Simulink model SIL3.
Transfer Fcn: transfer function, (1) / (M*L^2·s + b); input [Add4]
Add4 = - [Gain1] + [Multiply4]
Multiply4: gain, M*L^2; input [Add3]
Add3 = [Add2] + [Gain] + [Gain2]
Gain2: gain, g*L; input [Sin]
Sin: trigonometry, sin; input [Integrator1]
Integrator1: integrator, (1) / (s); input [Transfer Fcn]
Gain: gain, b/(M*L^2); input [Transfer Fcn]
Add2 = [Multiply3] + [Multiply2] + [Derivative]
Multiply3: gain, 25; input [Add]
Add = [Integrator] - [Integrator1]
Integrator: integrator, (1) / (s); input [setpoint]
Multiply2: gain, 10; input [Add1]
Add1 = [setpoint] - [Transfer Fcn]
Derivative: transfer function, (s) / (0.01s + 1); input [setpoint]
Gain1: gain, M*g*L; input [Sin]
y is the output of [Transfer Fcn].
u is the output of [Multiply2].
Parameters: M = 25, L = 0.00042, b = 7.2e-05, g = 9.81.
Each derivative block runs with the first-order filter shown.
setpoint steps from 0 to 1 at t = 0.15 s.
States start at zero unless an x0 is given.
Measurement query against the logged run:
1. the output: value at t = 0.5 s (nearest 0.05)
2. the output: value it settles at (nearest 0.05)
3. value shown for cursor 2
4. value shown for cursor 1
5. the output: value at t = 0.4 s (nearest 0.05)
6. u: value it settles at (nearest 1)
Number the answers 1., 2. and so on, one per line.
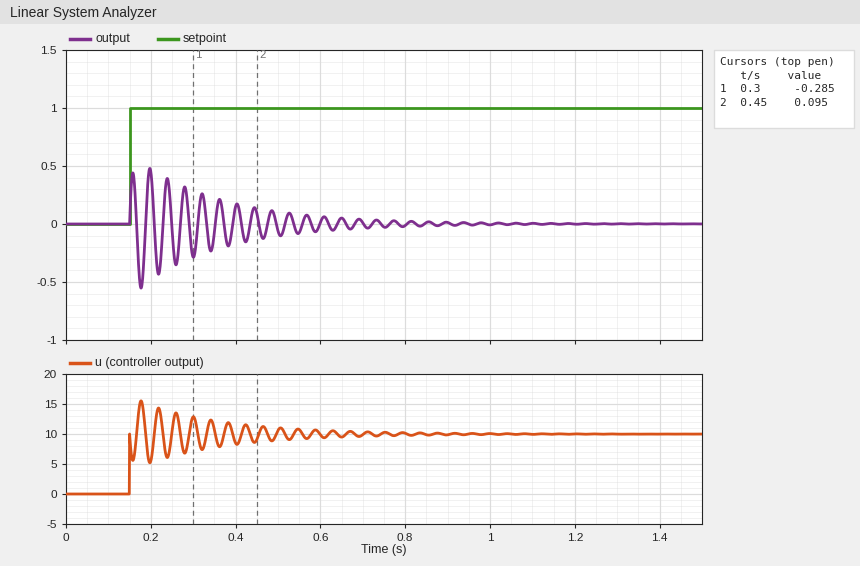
1. -0.05
2. 0.00
3. 0.095
4. -0.285
5. 0.15
6. 10
